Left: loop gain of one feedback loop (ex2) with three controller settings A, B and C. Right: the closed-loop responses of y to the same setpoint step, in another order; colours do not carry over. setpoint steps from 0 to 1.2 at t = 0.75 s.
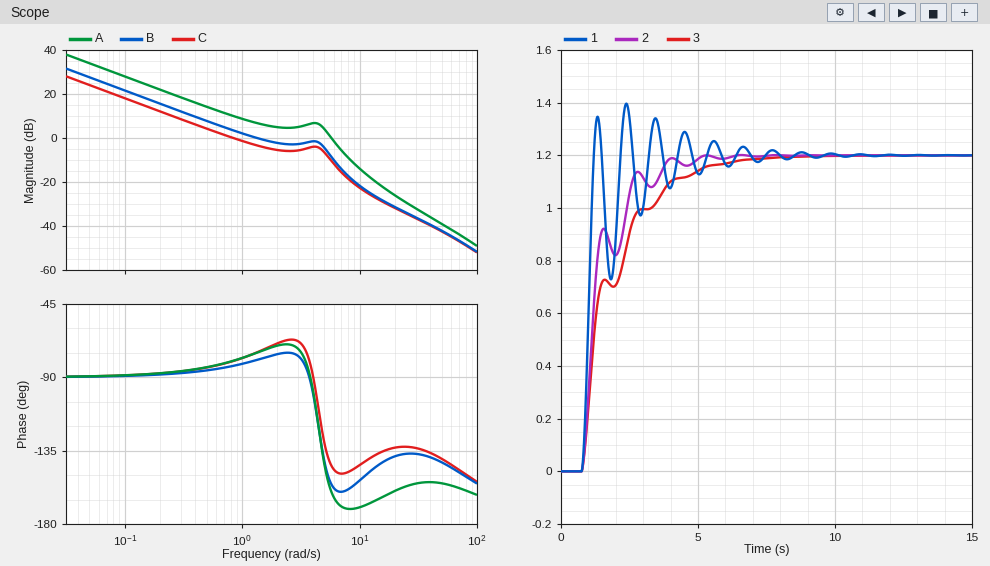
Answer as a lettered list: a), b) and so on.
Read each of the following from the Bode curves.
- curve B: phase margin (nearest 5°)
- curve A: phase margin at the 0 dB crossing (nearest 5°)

a) 100°
b) 20°
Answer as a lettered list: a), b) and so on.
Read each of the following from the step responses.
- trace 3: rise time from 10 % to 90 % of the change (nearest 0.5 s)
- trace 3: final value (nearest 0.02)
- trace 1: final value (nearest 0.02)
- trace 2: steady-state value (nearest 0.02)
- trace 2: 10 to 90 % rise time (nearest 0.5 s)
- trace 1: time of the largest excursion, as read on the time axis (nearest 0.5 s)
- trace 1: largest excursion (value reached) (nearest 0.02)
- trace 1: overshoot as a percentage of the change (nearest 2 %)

a) 3.0 s
b) 1.20
c) 1.20
d) 1.20
e) 1.5 s
f) 2.5 s
g) 1.40
h) 16 %
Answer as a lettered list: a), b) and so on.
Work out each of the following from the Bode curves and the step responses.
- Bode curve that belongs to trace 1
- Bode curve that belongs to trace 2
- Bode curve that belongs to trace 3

a) A
b) B
c) C
